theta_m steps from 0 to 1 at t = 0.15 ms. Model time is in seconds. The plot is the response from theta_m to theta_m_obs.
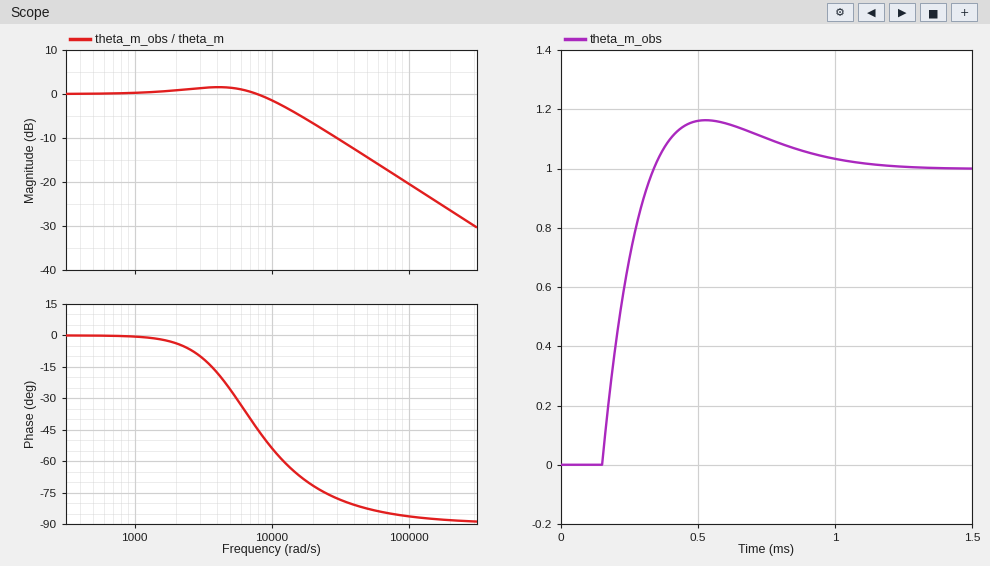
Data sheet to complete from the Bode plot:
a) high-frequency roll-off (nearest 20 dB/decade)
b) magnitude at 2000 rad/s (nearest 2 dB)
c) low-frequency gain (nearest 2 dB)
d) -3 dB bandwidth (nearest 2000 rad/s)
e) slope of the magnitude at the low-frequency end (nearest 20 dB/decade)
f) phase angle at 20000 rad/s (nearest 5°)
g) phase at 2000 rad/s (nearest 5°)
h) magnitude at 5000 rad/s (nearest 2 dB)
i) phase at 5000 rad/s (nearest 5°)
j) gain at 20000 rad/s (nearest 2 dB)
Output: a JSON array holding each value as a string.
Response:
["-20 dB/decade", "0 dB", "0 dB", "12000 rad/s", "0 dB/decade", "-70°", "-5°", "2 dB", "-25°", "-6 dB"]
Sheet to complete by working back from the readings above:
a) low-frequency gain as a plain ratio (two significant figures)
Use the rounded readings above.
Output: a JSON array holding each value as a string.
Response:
["1.0"]
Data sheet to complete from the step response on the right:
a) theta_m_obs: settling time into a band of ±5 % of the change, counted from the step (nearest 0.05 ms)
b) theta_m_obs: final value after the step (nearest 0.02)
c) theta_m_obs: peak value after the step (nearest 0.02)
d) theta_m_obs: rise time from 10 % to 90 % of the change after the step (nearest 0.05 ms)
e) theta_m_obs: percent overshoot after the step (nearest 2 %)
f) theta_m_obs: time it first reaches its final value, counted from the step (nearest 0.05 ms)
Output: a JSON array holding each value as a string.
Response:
["0.75 ms", "1.00", "1.16", "0.15 ms", "16 %", "0.20 ms"]
